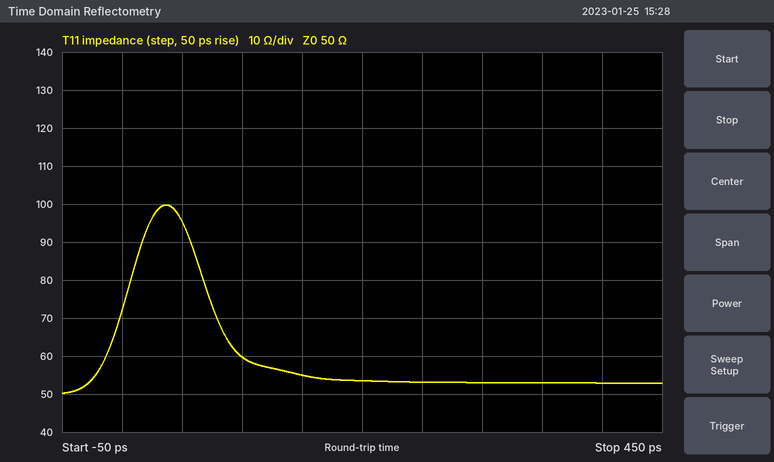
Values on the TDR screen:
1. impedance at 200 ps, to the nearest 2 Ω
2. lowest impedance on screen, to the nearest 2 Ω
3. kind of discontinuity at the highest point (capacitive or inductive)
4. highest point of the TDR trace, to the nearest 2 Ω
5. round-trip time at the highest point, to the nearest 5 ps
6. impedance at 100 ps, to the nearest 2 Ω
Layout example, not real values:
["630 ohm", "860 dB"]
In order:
["54 Ω", "50 Ω", "inductive", "100 Ω", "35 ps", "60 Ω"]
